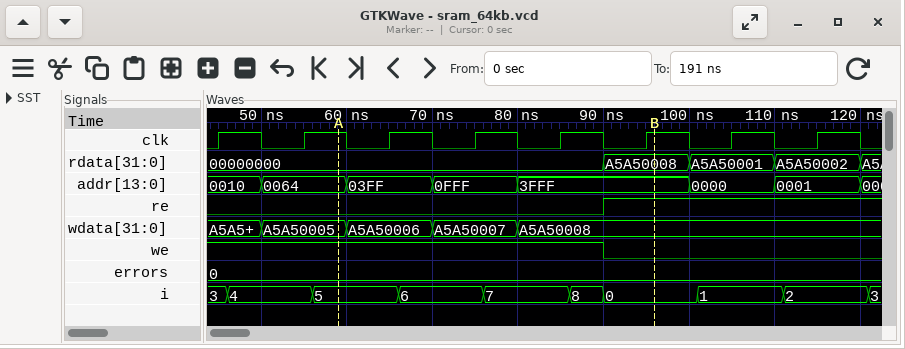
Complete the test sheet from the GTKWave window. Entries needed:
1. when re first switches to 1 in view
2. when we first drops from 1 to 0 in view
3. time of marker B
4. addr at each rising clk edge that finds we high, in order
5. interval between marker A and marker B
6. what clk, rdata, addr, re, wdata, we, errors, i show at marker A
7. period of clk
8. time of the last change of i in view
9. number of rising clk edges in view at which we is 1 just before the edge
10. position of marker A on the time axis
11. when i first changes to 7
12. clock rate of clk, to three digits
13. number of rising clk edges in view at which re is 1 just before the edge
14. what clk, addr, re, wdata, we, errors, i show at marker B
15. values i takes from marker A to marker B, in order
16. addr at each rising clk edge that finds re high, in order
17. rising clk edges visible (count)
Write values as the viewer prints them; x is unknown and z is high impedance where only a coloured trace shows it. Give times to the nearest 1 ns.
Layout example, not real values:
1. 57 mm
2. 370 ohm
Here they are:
1. 90 ns
2. 90 ns
3. 96 ns
4. 0010, 0064, 03FF, 0FFF, 3FFF
5. 37 ns
6. clk=1, rdata=00000000, addr=0064, re=0, wdata=A5A50005, we=1, errors=0, i=5
7. 10 ns
8. 121 ns
9. 5
10. 59 ns
11. 76 ns
12. 100 MHz
13. 3
14. clk=1, addr=3FFF, re=1, wdata=A5A50008, we=0, errors=0, i=0
15. 5, 6, 7, 8, 0
16. 3FFF, 0000, 0001
17. 8
